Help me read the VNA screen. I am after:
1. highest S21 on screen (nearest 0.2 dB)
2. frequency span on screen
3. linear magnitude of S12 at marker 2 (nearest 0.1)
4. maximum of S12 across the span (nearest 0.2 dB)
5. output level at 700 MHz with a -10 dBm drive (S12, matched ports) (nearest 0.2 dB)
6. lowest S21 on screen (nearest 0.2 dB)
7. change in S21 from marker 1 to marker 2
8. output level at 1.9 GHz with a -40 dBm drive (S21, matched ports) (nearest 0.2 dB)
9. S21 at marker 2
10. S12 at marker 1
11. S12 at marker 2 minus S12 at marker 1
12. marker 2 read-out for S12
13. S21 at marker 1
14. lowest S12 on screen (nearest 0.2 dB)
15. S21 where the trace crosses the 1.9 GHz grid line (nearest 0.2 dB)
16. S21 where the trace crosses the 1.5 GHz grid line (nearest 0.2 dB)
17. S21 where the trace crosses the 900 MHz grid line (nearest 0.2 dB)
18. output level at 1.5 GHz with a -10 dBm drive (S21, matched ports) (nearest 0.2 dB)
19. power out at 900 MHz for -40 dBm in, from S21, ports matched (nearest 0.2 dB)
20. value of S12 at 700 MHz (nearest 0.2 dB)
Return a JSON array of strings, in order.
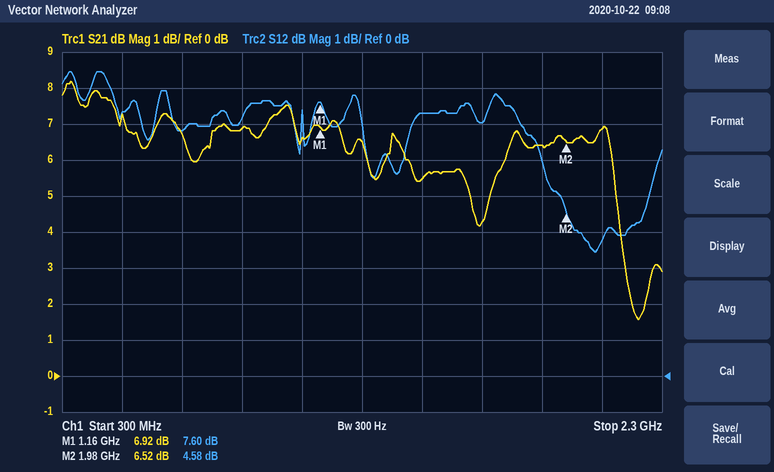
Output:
["8.2 dB", "2 GHz", "1.7", "8.4 dB", "-3.2 dBm", "1.6 dB", "-0.40 dB", "-33.6 dBm", "6.52 dB", "7.60 dB", "-3.02 dB", "4.58 dB", "6.92 dB", "3.4 dB", "6.4 dB", "5.4 dB", "6.8 dB", "-4.6 dBm", "-33.2 dBm", "6.8 dB"]
